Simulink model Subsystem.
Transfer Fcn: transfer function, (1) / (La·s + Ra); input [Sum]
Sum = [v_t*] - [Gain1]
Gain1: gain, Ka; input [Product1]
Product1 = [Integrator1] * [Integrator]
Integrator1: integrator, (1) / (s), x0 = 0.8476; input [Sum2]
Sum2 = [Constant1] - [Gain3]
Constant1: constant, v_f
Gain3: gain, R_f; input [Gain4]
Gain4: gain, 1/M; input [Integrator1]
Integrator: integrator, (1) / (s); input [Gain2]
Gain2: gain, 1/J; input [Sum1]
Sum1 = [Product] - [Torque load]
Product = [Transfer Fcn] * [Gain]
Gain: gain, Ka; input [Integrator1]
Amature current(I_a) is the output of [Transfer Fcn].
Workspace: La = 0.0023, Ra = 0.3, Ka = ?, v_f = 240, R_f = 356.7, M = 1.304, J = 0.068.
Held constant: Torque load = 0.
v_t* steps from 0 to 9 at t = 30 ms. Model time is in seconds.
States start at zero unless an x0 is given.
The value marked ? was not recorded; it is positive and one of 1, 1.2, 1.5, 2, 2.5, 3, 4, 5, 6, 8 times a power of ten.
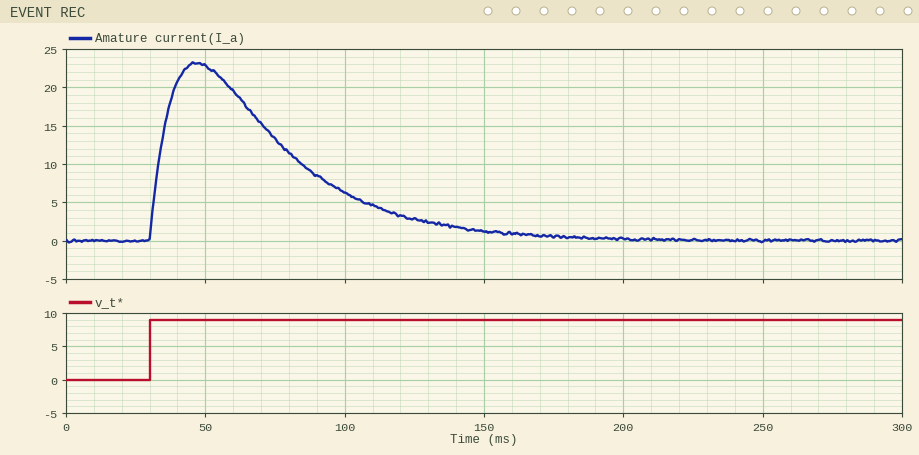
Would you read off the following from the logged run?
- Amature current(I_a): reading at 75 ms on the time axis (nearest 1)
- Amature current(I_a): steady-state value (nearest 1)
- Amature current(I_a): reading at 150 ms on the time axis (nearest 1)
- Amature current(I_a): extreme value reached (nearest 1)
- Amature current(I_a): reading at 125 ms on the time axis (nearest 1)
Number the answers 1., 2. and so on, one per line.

1. 13
2. 0
3. 1
4. 23
5. 3
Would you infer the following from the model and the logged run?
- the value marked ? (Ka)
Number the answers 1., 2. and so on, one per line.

1. 0.8
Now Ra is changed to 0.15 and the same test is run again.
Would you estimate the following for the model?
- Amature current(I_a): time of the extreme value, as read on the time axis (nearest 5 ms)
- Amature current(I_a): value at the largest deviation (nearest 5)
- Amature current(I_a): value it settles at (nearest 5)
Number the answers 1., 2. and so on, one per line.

1. 50 ms
2. 35
3. 0
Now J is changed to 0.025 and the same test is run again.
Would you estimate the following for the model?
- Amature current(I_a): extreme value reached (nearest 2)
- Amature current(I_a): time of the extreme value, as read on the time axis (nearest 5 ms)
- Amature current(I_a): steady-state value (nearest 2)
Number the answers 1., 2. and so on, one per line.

1. 20
2. 40 ms
3. 0
